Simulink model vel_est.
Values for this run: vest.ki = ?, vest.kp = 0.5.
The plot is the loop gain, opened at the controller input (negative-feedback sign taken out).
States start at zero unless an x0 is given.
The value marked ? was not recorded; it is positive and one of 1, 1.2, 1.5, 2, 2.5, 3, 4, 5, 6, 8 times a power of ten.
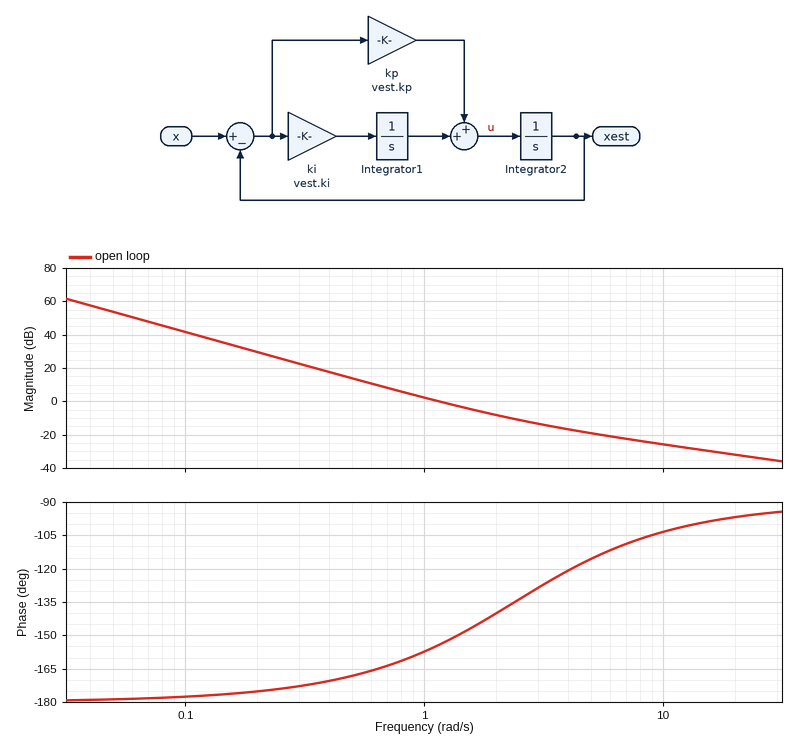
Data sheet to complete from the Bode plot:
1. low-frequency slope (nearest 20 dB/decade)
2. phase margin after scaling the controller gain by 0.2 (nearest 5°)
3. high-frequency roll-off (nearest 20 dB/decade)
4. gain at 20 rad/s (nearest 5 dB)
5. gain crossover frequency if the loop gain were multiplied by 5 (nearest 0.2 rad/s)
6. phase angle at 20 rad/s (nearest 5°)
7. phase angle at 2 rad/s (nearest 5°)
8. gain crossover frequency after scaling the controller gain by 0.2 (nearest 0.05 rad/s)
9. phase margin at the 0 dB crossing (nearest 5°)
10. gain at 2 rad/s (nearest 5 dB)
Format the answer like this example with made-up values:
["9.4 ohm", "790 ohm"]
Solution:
["-40 dB/decade", "10°", "-20 dB/decade", "-30 dB", "3.2 rad/s", "-95°", "-140°", "0.50 rad/s", "25°", "-10 dB"]
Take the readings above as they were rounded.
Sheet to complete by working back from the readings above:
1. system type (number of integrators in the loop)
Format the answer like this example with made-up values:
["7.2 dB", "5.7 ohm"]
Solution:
["2"]
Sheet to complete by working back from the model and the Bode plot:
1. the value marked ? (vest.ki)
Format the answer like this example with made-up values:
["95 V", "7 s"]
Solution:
["1.2"]
